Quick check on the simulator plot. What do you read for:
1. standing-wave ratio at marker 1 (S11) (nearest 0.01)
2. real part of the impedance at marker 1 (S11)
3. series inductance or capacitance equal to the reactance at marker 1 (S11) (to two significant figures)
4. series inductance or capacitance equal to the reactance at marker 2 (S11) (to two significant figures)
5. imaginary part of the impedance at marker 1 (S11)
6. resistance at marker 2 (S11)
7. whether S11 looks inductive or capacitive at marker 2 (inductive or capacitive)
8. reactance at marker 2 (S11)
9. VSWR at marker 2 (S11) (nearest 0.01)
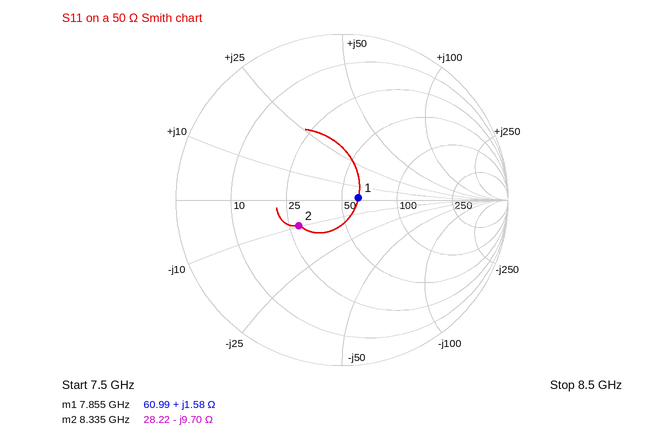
1.22
60.99 Ω
32 pH
2.0 pF
+1.58 Ω
28.22 Ω
capacitive
-9.70 Ω
1.87
